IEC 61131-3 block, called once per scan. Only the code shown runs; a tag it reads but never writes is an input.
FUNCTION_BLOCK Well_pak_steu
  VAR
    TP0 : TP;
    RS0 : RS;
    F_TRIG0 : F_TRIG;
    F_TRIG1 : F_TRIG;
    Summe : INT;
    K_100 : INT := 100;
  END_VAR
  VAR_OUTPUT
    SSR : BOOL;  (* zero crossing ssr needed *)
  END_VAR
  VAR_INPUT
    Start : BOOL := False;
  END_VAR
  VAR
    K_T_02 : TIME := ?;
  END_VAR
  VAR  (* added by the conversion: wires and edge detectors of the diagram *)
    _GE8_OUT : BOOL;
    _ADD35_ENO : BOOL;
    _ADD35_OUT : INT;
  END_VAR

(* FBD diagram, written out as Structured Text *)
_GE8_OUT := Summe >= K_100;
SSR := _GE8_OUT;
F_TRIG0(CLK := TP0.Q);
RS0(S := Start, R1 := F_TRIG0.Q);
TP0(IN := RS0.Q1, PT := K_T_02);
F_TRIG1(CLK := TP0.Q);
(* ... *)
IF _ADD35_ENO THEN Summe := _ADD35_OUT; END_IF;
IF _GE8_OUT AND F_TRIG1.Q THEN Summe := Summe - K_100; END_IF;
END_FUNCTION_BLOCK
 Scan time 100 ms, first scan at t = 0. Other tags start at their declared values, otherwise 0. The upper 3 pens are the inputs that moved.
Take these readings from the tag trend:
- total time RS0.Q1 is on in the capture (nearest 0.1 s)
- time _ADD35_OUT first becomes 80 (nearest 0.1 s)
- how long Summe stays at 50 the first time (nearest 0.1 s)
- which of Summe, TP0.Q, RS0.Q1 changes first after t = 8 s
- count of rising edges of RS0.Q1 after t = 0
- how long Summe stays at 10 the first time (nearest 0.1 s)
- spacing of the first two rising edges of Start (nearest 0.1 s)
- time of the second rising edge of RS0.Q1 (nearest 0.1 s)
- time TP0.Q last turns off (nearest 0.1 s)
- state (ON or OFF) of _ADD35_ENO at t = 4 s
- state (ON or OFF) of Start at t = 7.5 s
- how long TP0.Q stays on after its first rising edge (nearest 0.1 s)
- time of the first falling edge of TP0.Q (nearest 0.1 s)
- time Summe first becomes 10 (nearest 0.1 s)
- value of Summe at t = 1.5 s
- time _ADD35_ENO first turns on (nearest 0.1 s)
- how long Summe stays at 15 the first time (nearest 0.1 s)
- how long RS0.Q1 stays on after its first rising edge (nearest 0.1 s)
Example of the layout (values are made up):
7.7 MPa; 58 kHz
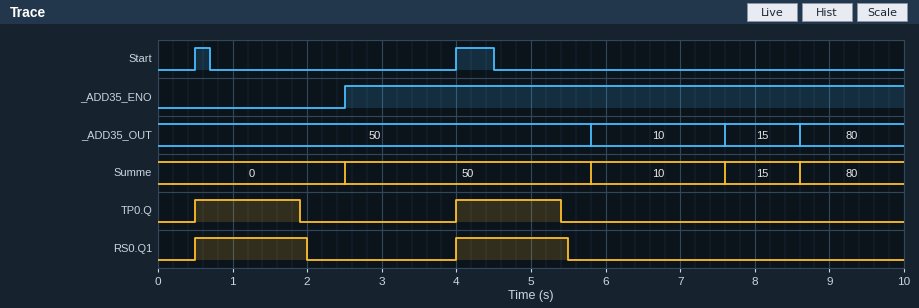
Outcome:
3.0 s; 8.6 s; 3.3 s; Summe; 2; 1.8 s; 3.5 s; 4.0 s; 5.4 s; ON; OFF; 1.4 s; 1.9 s; 5.8 s; 0; 2.5 s; 1.0 s; 1.5 s
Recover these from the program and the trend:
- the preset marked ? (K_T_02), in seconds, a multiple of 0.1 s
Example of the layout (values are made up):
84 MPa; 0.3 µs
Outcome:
1.4 s
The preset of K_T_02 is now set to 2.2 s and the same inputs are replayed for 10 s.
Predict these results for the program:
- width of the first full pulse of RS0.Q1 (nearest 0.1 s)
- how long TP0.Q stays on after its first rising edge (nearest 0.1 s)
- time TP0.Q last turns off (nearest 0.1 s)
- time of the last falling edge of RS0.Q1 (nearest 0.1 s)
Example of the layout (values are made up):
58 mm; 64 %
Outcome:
2.3 s; 2.2 s; 6.2 s; 6.3 s
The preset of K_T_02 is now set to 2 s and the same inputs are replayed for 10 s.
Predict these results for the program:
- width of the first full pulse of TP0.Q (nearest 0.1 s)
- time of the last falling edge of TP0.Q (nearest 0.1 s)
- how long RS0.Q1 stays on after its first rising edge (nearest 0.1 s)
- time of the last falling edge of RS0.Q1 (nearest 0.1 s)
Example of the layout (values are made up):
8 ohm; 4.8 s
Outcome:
2.0 s; 6.0 s; 2.1 s; 6.1 s
